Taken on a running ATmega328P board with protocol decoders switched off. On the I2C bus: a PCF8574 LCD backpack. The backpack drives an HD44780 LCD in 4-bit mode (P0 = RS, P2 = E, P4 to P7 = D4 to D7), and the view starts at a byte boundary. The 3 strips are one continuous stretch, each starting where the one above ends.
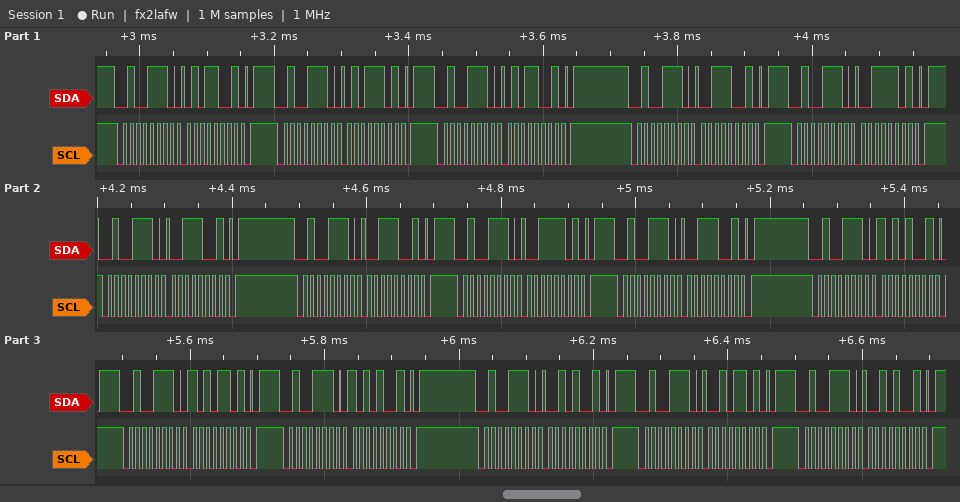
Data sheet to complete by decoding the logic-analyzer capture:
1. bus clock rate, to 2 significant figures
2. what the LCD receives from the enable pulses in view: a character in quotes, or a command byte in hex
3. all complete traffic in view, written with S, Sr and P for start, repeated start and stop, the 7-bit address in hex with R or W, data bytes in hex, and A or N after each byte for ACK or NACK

100 kHz
'S' ':'
S 27W A 59 A P S 27W A 5D A P S 27W A 59 A P S 27W A 39 A P S 27W A 3D A P S 27W A 39 A P S 27W A 39 A P S 27W A 3D A P S 27W A 39 A P S 27W A A9 A P S 27W A AD A P S 27W A A9 A P S 27W A 29 A P S 27W A 2D A P S 27W A 29 A P
